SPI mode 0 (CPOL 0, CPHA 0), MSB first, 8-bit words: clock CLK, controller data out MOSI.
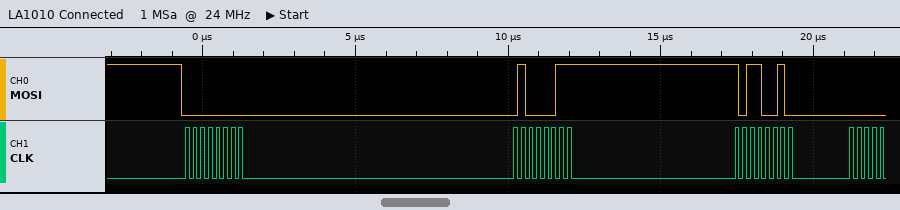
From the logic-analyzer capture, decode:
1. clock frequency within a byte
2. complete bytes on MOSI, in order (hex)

4 MHz
00 43 B2
